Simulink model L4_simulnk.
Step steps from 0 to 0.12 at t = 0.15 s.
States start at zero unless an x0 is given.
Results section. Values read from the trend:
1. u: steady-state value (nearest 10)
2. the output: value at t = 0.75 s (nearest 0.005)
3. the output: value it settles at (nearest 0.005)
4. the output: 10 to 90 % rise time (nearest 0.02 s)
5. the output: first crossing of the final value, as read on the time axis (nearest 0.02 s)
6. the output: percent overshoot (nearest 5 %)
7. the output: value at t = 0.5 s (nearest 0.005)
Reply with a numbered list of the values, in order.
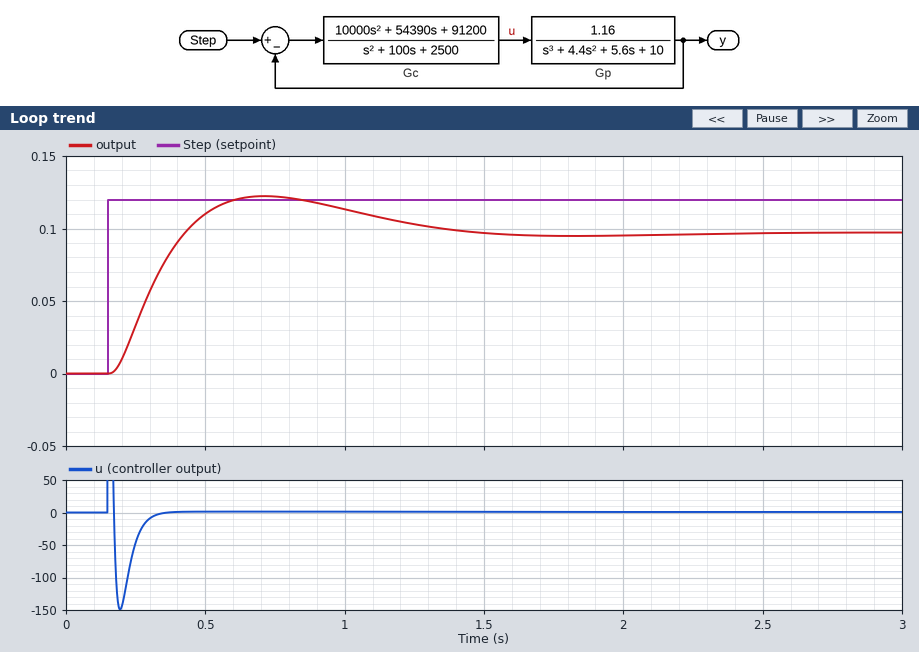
1. 0
2. 0.120
3. 0.095
4. 0.18 s
5. 0.42 s
6. 25 %
7. 0.110
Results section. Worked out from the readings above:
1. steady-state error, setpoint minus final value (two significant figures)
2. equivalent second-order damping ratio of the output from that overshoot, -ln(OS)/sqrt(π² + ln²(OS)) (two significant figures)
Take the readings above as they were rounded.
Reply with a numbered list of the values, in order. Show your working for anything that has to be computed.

1. 0.12 - 0.095 = 0.025
2. ln(0.25) = -1.386; 1.386 / sqrt(9.870 + 1.922) = 0.40
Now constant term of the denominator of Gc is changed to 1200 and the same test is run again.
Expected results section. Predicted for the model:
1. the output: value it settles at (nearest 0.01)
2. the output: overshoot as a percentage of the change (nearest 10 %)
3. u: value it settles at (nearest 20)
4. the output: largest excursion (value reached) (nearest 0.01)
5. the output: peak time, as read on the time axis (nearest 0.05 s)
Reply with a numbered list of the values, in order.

1. 0.11
2. 40 %
3. 0
4. 0.15
5. 0.50 s
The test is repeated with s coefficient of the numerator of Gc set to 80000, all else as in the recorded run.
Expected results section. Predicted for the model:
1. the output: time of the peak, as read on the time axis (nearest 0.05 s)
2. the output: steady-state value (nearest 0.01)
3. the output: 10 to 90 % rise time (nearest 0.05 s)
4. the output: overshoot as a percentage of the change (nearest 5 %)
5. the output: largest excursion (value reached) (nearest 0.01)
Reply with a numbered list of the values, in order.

1. 0.60 s
2. 0.10
3. 0.15 s
4. 35 %
5. 0.13
